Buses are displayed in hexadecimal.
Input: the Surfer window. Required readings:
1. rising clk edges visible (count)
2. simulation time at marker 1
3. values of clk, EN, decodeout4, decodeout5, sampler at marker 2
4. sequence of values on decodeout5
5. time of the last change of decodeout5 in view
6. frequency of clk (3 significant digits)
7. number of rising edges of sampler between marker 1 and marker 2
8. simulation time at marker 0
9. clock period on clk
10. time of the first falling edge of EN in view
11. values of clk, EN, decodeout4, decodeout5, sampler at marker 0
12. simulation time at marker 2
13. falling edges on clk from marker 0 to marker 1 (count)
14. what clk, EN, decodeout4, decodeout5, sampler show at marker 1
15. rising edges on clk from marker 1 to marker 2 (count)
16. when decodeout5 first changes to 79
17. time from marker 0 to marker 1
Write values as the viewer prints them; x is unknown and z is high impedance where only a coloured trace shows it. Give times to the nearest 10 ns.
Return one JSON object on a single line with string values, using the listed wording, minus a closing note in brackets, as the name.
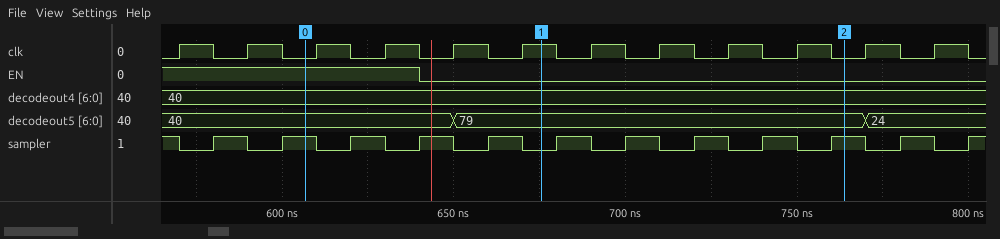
{"rising clk edges visible": "12", "simulation time at marker 1": "680 ns", "values of clk, EN, decodeout4, decodeout5, sampler at marker 2": "clk=0, EN=0, decodeout4=40, decodeout5=79, sampler=1", "sequence of values on decodeout5": "40, 79, 24", "time of the last change of decodeout5 in view": "770 ns", "frequency of clk": "50.0 MHz", "number of rising edges of sampler between marker 1 and marker 2": "5", "simulation time at marker 0": "610 ns", "clock period on clk": "20 ns", "time of the first falling edge of EN in view": "640 ns", "values of clk, EN, decodeout4, decodeout5, sampler at marker 0": "clk=0, EN=1, decodeout4=40, decodeout5=40, sampler=1", "simulation time at marker 2": "760 ns", "falling edges on clk from marker 0 to marker 1": "3", "what clk, EN, decodeout4, decodeout5, sampler show at marker 1": "clk=1, EN=0, decodeout4=40, decodeout5=79, sampler=0", "rising edges on clk from marker 1 to marker 2": "4", "when decodeout5 first changes to 79": "650 ns", "time from marker 0 to marker 1": "70 ns"}
